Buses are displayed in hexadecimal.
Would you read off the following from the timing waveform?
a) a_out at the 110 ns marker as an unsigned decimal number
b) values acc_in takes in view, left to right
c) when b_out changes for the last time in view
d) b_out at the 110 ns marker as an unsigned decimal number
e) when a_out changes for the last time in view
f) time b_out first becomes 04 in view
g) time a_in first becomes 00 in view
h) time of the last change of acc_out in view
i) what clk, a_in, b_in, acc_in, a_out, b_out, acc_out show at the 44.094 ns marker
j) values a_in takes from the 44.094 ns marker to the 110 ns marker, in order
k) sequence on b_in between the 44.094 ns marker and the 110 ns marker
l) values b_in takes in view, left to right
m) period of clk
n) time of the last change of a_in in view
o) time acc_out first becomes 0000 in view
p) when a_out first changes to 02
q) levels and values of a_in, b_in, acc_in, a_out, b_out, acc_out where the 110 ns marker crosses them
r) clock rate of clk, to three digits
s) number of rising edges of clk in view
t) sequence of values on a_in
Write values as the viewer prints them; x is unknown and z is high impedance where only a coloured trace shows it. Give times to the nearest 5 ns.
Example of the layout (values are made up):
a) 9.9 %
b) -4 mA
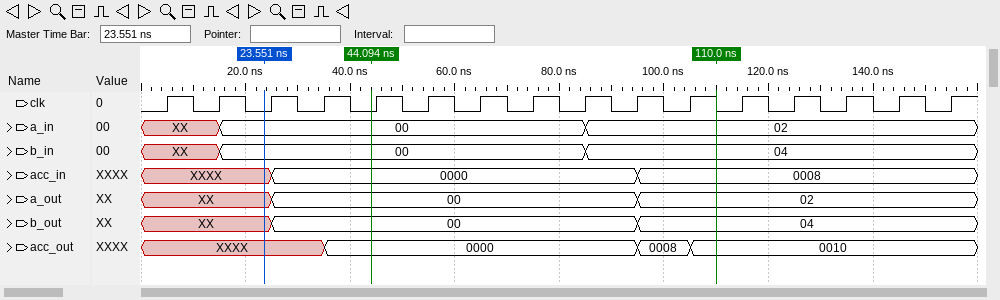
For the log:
a) 2
b) XXXX, 0000, 0008
c) 95 ns
d) 4
e) 95 ns
f) 95 ns
g) 15 ns
h) 105 ns
i) clk=0, a_in=00, b_in=00, acc_in=0000, a_out=00, b_out=00, acc_out=0000
j) 00, 02
k) 00, 04
l) XX, 00, 04
m) 10 ns
n) 85 ns
o) 35 ns
p) 95 ns
q) a_in=02, b_in=04, acc_in=0008, a_out=02, b_out=04, acc_out=0010
r) 100 MHz
s) 16
t) XX, 00, 02
